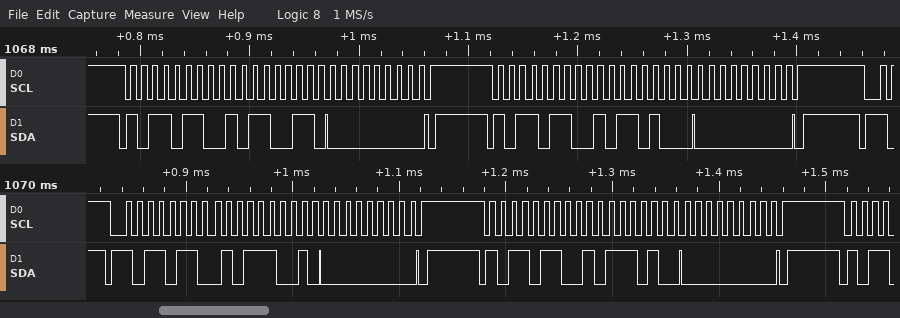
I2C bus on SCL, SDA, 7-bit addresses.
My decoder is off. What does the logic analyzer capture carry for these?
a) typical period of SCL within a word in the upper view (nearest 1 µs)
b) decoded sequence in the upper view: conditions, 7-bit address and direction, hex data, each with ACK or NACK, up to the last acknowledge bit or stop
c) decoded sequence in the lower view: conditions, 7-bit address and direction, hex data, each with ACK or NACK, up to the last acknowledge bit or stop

10 µs
start, address 5B write ACK, B3 ACK, 00 ACK, stop, start, address 5B write ACK, B4 ACK, 00 ACK, stop
start, address 5B write ACK, B9 ACK, 00 ACK, stop, start, address 5B write ACK, BA ACK, 00 ACK, stop
